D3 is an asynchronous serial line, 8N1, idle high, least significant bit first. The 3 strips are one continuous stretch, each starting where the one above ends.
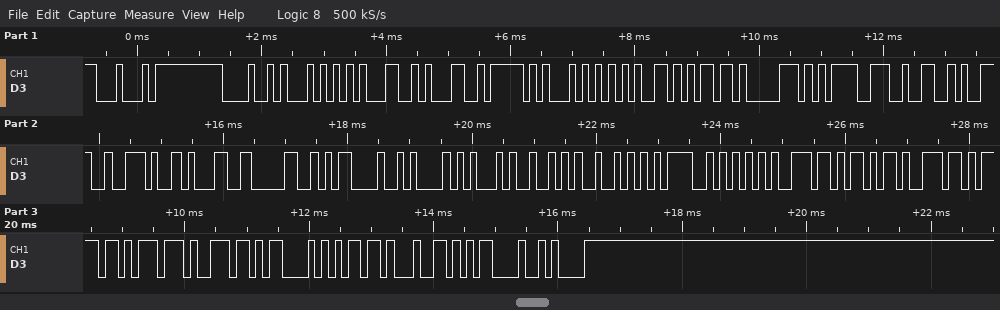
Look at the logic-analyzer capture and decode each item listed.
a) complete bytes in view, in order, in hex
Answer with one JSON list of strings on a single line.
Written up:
["44 48 54 31 31 5F 54 65 6D 70 3D 32 39 2E 31 30 0D 0A 45 52 52 3D 55 6E 6B 6E 6F 77 6E 43 6D 64 0D 0A"]
